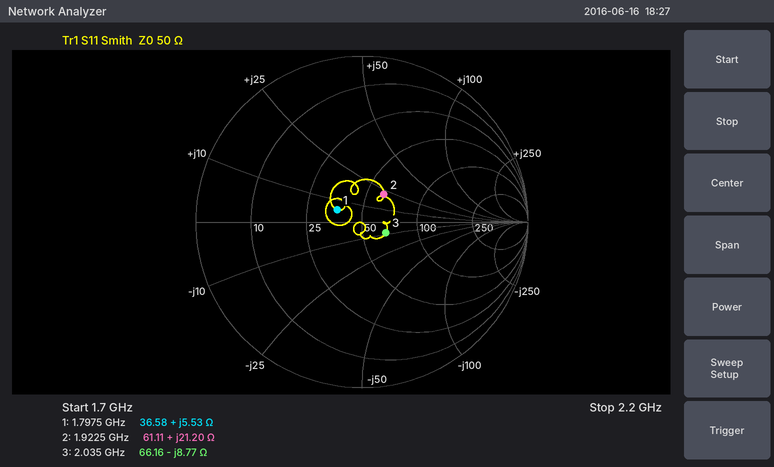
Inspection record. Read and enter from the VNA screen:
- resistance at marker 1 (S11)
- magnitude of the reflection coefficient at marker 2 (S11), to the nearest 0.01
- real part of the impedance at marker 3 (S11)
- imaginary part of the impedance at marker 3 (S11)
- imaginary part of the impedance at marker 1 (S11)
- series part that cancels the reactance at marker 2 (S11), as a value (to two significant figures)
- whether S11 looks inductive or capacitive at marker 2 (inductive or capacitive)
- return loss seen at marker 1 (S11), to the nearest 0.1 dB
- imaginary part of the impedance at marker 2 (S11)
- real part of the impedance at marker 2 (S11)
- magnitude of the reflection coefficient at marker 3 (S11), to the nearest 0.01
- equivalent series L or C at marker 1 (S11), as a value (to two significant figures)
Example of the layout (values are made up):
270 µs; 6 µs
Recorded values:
36.58 Ω; 0.21; 66.16 Ω; -8.77 Ω; +5.53 Ω; 3.9 pF; inductive; 15.5 dB; +21.20 Ω; 61.11 Ω; 0.16; 490 pH
